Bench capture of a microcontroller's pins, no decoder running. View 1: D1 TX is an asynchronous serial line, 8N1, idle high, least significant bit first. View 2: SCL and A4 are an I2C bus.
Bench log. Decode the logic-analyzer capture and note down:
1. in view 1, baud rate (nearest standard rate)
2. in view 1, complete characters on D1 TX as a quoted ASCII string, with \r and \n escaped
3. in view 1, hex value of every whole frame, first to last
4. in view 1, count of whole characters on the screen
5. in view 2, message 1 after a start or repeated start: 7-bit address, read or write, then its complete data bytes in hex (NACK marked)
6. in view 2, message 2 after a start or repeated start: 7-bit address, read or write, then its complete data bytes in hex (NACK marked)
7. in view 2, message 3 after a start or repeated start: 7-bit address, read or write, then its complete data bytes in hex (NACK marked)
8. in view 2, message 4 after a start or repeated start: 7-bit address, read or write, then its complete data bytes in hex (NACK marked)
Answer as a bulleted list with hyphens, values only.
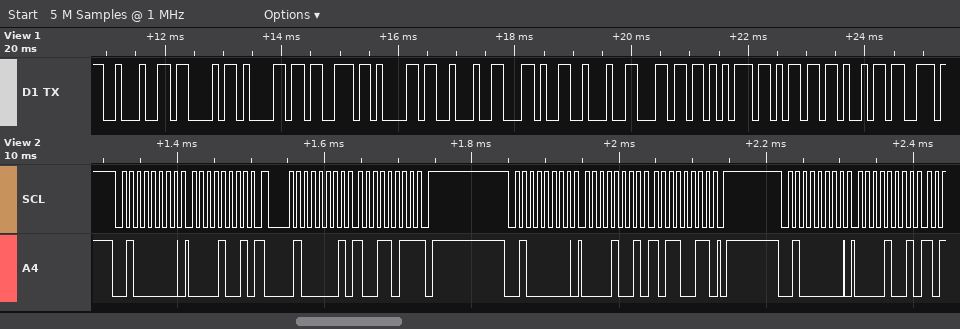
- 9600 baud
- "\"Casa\",\"lumi"
- 22 43 61 73 61 22 2C 22 6C 75 6D 69
- 12
- 0x20 write: 09
- 0x20 read: 9B NACK
- 0x20 write: 09 B3
- 0x20 write: 09
